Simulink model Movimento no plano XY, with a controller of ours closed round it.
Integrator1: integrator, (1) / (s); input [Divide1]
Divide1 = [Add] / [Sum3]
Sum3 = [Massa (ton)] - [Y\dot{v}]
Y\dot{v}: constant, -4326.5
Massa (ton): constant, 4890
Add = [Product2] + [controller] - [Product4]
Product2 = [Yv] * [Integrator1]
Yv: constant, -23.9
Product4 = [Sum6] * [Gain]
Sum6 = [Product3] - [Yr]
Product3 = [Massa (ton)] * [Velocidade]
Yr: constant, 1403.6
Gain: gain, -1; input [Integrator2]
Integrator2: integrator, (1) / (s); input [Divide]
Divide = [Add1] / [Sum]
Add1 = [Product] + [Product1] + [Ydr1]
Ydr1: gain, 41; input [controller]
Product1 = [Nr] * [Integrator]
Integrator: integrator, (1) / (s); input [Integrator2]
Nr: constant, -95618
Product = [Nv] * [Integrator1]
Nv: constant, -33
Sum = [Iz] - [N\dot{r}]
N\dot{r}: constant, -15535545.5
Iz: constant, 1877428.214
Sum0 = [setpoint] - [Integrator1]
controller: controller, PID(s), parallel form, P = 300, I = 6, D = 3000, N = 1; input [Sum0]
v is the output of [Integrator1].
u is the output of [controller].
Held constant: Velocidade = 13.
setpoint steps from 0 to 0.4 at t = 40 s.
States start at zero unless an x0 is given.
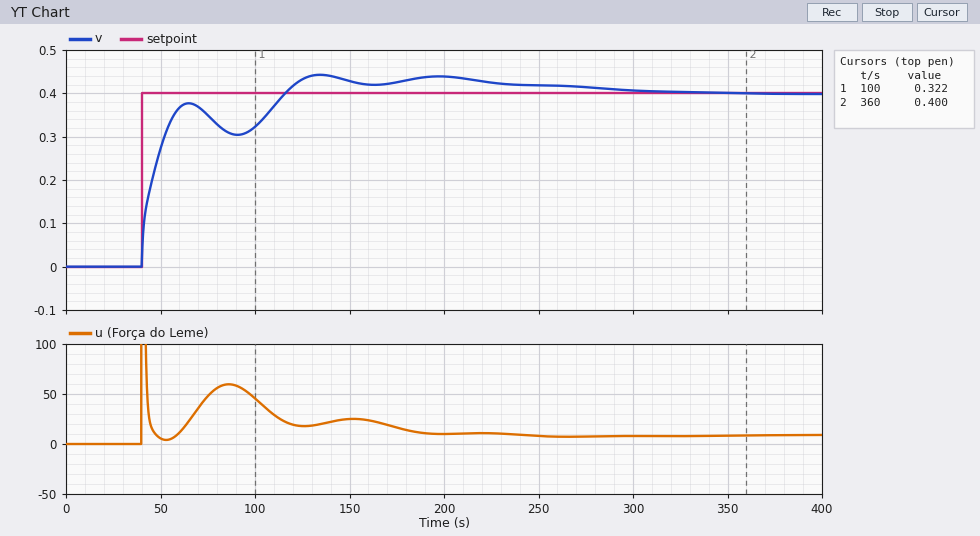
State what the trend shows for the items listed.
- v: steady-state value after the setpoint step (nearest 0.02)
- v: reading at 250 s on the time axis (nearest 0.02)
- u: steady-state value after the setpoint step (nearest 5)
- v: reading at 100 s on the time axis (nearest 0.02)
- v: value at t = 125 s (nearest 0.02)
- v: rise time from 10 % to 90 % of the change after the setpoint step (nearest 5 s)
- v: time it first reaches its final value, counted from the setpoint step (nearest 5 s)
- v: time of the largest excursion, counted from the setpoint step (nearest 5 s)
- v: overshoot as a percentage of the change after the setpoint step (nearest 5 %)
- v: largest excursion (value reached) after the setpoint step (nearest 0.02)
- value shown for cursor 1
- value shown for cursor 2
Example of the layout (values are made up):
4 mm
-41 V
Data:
0.40
0.42
10
0.32
0.44
20 s
75 s
95 s
10 %
0.44
0.322
0.400
